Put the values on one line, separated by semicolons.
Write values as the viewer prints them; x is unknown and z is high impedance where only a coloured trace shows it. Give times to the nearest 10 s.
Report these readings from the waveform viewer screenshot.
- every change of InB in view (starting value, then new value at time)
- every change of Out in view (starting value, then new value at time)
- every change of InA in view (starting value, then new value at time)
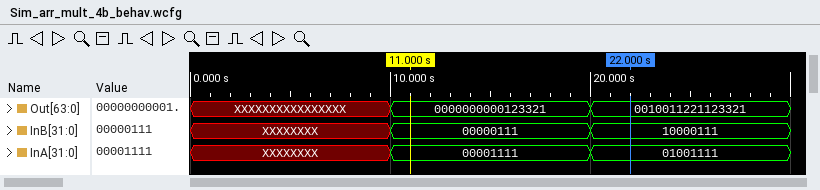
XXXXXXXX, 00000111 at 10 s, 10000111 at 20 s; XXXXXXXXXXXXXXXX, 0000000000123321 at 10 s, 0010011221123321 at 20 s; XXXXXXXX, 00001111 at 10 s, 01001111 at 20 s
